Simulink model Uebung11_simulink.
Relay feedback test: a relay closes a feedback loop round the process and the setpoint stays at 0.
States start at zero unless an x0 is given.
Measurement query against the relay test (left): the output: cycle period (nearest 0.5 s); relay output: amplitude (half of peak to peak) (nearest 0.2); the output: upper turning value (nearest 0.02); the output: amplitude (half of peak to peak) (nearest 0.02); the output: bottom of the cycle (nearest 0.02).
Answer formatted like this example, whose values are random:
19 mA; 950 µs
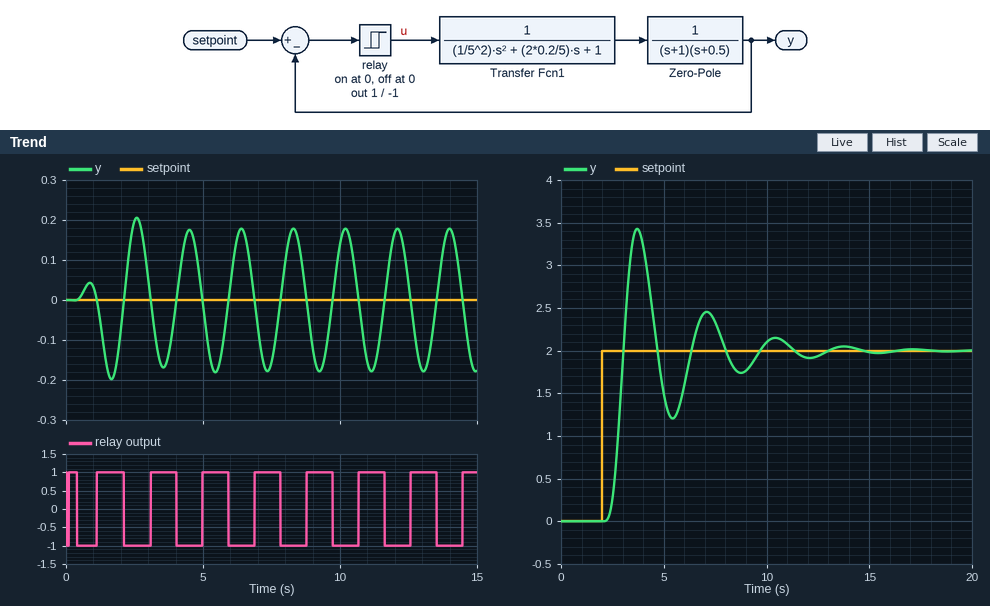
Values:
2.0 s; 1.0; 0.18; 0.18; -0.18
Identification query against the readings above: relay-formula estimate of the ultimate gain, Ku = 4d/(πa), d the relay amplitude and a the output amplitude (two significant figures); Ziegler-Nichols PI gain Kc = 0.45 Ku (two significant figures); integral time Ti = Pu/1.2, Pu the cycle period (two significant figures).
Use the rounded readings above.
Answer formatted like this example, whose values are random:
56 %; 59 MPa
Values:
7.1; 3.2; 1.7 s
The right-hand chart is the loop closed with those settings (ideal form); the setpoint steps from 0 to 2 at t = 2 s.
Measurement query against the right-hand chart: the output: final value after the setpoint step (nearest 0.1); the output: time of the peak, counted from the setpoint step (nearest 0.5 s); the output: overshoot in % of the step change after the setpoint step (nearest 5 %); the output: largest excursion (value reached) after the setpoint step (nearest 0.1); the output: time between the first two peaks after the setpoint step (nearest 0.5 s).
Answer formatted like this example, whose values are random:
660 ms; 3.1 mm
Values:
2.0; 1.5 s; 70 %; 3.4; 3.5 s
